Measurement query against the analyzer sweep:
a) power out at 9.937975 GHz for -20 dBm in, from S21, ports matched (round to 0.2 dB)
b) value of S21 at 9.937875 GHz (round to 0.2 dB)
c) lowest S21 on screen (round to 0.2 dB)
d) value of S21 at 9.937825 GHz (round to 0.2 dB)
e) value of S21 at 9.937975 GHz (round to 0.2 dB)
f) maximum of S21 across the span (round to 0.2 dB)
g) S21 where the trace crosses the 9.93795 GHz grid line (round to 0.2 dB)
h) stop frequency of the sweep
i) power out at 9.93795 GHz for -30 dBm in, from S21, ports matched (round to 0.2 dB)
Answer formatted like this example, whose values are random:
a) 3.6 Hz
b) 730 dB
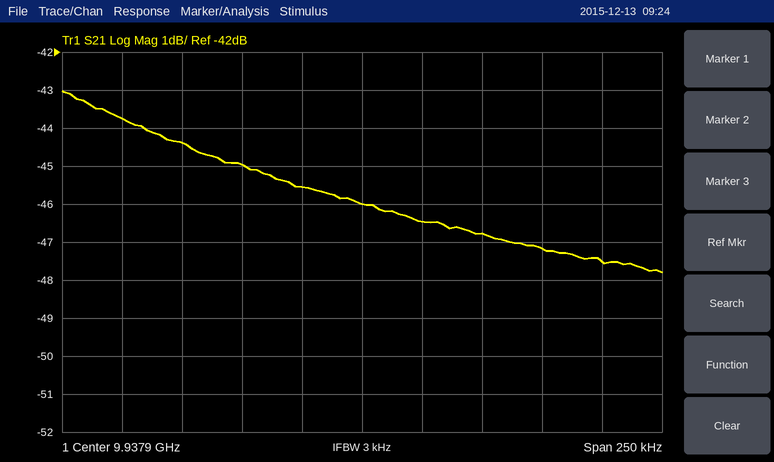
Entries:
a) -67.2 dBm
b) -45.6 dB
c) -47.8 dB
d) -44.4 dB
e) -47.2 dB
f) -43.0 dB
g) -46.8 dB
h) 9.938025 GHz
i) -76.8 dBm
